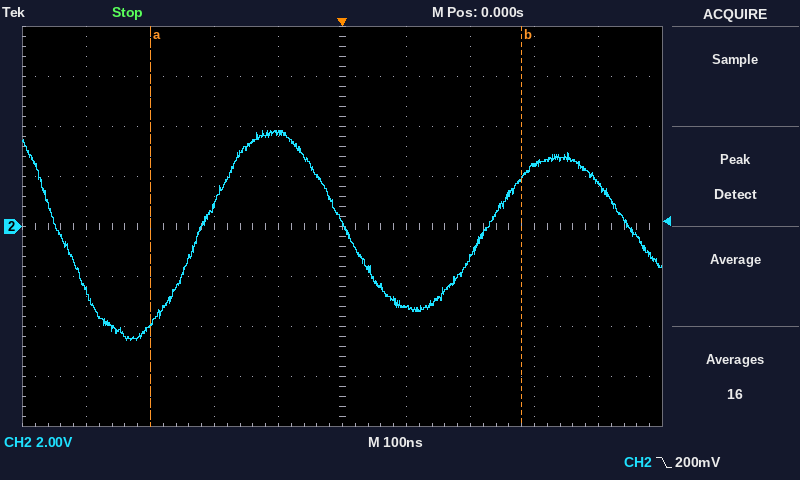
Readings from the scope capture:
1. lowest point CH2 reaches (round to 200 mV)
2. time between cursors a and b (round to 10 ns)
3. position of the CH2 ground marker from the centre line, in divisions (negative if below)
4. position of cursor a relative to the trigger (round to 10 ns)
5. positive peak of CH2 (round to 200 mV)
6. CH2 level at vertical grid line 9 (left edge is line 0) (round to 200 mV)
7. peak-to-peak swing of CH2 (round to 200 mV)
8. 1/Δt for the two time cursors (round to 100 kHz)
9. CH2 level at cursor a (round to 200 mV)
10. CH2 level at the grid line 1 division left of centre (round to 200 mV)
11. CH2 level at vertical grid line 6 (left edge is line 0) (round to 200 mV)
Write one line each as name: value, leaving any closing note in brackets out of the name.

lowest point CH2 reaches: -4.6 V
time between cursors a and b: 580 ns
position of the CH2 ground marker from the centre line, in divisions: 0.0 div
position of cursor a relative to the trigger: -300 ns
positive peak of CH2: 3.8 V
CH2 level at vertical grid line 9 (left edge is line 0): 1.8 V
peak-to-peak swing of CH2: 8.4 V
1/Δt for the two time cursors: 1.7 MHz
CH2 level at cursor a: -3.8 V
CH2 level at the grid line 1 division left of centre: 3.8 V
CH2 level at vertical grid line 6 (left edge is line 0): -3.2 V
